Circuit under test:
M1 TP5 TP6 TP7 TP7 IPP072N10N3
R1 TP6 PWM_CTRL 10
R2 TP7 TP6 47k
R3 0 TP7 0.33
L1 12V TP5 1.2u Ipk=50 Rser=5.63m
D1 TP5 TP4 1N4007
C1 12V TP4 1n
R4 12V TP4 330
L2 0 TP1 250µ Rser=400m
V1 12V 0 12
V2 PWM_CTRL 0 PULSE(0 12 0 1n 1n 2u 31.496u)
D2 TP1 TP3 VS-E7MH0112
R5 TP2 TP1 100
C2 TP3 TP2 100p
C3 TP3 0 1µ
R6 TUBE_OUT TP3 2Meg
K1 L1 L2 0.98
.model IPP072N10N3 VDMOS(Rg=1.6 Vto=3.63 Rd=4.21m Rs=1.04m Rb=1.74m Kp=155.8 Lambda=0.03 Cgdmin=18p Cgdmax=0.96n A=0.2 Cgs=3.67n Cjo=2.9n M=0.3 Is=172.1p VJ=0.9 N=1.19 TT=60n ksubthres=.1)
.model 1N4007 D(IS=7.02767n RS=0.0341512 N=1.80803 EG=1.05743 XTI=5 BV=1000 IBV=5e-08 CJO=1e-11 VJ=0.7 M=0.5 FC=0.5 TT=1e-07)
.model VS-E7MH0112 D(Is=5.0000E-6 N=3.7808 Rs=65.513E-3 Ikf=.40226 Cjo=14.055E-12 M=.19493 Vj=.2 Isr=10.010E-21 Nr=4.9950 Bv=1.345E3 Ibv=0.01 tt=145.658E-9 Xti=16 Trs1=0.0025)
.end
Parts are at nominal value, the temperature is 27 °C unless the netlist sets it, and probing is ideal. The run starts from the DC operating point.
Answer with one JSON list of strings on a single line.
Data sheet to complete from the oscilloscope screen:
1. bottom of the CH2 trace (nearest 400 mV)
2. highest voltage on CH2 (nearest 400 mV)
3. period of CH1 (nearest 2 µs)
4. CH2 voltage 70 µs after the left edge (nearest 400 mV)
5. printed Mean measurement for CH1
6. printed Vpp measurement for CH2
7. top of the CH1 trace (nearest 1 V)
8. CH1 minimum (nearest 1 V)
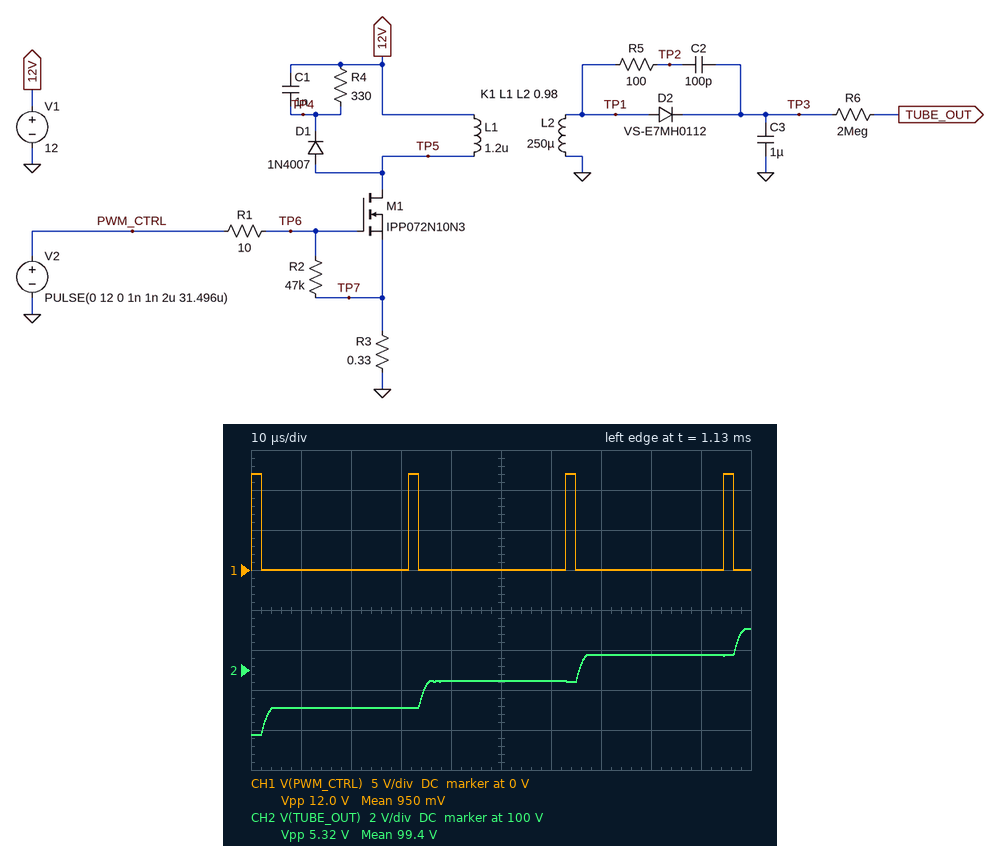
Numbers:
["96.8 V", "102.0 V", "32 µs", "100.8 V", "950 mV", "5.32 V", "12 V", "0 V"]
